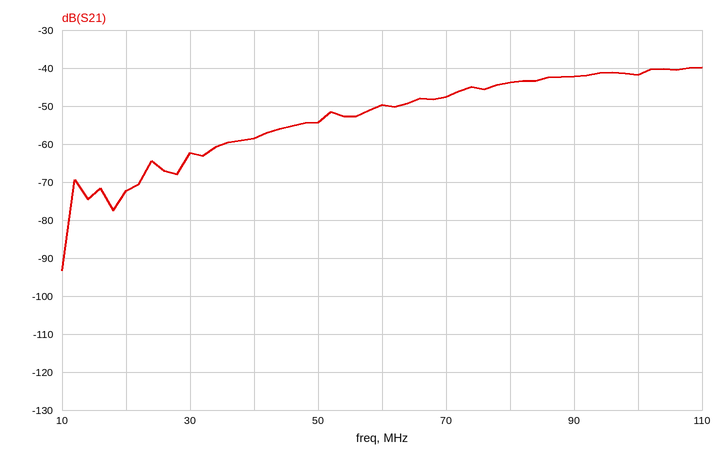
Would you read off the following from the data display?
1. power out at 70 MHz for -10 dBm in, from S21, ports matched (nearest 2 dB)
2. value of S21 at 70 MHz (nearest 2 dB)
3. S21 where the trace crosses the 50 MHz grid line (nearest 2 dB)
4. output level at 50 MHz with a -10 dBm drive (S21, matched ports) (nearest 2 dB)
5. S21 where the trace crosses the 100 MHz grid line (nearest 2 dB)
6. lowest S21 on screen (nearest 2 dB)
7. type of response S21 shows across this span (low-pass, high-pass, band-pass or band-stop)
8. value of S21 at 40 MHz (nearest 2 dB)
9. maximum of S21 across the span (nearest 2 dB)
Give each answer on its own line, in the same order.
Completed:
-58 dBm
-48 dB
-54 dB
-64 dBm
-42 dB
-94 dB
high-pass
-58 dB
-40 dB
